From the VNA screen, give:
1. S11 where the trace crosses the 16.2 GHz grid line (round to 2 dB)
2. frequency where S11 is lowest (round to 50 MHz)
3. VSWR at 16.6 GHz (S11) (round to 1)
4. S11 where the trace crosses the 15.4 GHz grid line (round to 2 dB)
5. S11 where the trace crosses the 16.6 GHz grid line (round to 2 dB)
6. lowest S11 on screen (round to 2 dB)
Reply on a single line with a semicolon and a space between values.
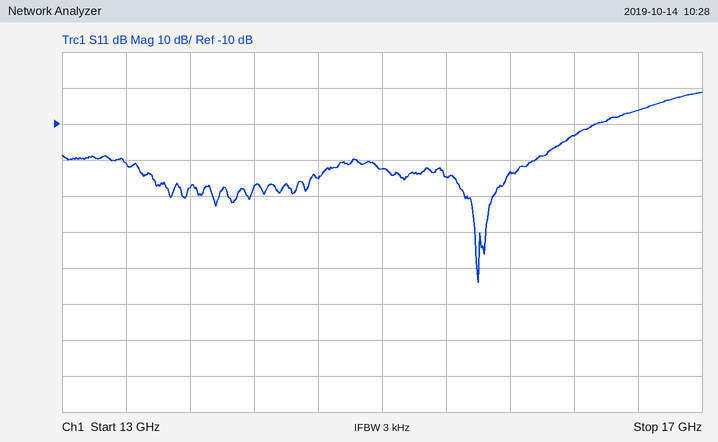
-14 dB; 15.60 GHz; 3; -24 dB; -6 dB; -54 dB
